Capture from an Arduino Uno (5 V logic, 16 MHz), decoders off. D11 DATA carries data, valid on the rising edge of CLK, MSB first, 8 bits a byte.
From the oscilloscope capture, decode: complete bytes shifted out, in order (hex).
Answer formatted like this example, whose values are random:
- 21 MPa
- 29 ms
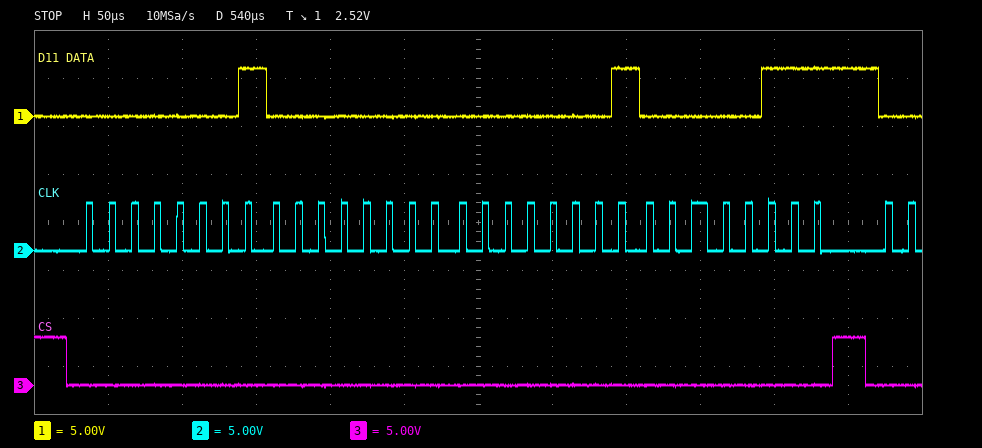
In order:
- 01 00 01 07
